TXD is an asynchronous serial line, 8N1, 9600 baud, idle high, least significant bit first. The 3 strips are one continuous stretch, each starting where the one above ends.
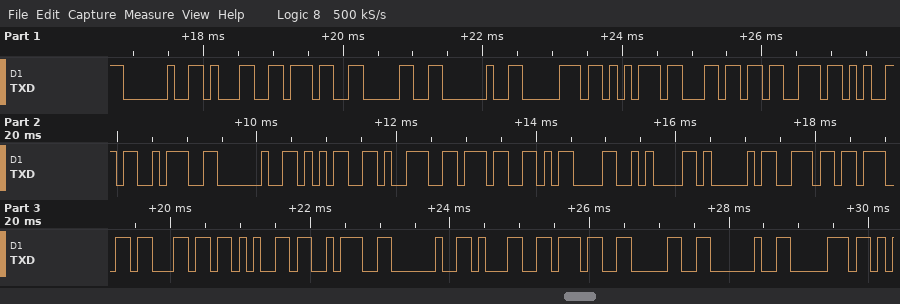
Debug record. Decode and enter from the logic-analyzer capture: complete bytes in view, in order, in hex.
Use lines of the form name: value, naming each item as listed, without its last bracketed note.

complete bytes in view, in order, in hex: 20 31 37 30 20 70 75 6C 73 65 3A 20 35 39 37 0D 0A 41 6E 67 6C 65 3A 20 31 37 30 20 70
